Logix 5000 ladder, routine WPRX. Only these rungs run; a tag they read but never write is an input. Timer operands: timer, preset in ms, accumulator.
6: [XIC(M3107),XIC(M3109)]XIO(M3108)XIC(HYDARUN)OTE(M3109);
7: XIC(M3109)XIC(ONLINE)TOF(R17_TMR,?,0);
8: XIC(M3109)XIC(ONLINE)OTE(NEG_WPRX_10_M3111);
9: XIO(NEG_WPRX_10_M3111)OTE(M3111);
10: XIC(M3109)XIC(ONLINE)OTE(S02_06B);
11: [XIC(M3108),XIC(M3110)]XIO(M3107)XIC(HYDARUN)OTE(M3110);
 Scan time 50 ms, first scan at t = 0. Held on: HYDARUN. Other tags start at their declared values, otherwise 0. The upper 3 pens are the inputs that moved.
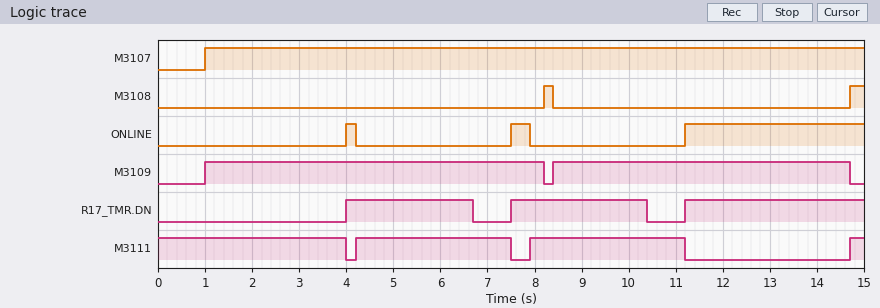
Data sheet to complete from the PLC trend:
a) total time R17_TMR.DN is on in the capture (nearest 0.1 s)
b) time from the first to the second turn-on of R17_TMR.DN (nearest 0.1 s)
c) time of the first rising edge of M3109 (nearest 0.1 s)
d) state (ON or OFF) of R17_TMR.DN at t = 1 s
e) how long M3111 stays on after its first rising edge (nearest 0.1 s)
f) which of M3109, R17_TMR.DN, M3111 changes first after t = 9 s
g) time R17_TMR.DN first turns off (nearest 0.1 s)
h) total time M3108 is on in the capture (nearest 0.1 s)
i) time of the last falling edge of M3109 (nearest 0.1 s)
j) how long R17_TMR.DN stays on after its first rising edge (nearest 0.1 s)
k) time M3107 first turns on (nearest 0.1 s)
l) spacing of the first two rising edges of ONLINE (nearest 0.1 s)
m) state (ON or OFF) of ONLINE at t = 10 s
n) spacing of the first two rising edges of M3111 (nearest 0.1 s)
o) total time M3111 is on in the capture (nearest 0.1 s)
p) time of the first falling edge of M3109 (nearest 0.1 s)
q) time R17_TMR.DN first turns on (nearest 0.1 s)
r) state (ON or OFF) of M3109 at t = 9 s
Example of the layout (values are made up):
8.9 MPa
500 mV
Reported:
9.4 s
3.5 s
1.0 s
OFF
3.3 s
R17_TMR.DN
6.7 s
0.5 s
14.7 s
2.7 s
1.0 s
3.5 s
OFF
3.7 s
10.9 s
8.2 s
4.0 s
ON
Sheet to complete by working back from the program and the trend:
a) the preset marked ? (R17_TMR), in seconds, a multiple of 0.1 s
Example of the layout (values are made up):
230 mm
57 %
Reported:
2.5 s
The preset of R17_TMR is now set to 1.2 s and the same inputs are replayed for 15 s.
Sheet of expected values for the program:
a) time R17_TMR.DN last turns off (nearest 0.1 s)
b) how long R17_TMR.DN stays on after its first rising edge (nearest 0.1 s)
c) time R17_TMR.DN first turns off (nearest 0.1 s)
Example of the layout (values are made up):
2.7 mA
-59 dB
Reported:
9.1 s
1.4 s
5.4 s
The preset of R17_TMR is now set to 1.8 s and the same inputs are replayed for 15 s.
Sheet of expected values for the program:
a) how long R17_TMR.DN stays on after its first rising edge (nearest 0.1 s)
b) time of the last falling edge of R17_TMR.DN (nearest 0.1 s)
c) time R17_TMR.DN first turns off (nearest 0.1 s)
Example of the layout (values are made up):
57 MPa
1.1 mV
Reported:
2.0 s
9.7 s
6.0 s
